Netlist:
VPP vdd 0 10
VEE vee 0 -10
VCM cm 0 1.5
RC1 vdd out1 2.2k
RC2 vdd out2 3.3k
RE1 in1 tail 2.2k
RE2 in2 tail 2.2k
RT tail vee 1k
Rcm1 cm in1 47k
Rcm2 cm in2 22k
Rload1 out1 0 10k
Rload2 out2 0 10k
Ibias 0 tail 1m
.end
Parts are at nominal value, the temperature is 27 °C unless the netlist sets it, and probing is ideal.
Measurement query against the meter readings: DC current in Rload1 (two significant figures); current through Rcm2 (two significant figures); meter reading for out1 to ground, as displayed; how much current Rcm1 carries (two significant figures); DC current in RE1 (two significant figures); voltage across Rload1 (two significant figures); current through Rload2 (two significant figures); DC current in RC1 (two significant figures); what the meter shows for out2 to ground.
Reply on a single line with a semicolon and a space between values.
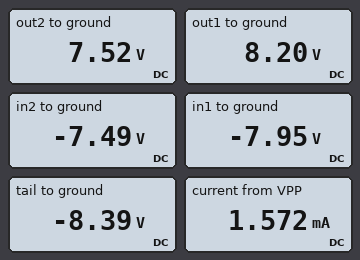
820 µA; 410 µA; 8.20 V; 200 µA; 200 µA; 8.2 V; 750 µA; 820 µA; 7.52 V
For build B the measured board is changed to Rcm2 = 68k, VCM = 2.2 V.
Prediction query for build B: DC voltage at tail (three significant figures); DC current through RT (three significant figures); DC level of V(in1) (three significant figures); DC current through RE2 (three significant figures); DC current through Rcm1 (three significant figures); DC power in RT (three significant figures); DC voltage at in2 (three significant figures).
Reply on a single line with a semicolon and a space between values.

-8.63 V; 1.37 mA; -8.14 V; 154 µA; 220 µA; 1.89 mW; -8.29 V
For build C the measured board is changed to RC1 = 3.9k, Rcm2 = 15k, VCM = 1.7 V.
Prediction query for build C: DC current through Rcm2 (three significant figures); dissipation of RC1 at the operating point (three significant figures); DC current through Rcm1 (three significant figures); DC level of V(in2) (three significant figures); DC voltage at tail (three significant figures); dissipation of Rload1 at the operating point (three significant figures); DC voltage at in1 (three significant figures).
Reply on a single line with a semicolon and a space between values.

577 µA; 2.02 mW; 202 µA; -6.95 V; -8.22 V; 5.18 mW; -7.78 V
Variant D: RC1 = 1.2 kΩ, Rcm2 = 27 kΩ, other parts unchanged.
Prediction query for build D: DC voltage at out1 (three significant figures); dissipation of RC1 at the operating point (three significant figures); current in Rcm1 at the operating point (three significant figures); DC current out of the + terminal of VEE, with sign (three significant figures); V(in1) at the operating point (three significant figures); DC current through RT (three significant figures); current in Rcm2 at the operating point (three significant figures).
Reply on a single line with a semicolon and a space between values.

8.93 V; 957 µW; 202 µA; -1.54 mA; -8.01 V; 1.54 mA; 341 µA
